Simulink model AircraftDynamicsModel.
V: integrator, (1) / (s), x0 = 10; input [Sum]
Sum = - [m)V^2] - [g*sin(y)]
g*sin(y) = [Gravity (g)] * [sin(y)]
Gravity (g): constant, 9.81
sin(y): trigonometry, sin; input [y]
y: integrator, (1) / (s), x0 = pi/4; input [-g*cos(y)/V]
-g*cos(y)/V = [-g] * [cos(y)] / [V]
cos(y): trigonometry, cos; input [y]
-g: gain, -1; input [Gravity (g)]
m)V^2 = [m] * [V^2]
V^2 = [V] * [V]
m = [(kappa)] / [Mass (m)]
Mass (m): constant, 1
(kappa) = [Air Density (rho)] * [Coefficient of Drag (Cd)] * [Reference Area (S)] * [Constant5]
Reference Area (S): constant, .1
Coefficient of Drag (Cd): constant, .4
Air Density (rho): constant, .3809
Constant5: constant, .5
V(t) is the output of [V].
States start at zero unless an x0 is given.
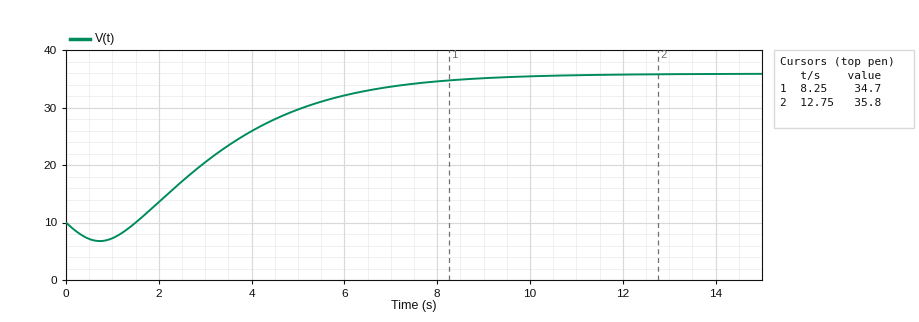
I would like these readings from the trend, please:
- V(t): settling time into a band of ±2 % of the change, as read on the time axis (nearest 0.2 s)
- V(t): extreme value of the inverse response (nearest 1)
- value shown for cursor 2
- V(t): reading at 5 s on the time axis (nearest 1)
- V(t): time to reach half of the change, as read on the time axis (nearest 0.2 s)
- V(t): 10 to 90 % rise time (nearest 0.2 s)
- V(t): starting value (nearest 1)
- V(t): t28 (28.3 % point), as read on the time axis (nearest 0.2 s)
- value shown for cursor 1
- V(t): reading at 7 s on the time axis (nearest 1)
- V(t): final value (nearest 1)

9.8 s
7
35.8
30
3.4 s
4.8 s
10
2.6 s
34.7
34
36
